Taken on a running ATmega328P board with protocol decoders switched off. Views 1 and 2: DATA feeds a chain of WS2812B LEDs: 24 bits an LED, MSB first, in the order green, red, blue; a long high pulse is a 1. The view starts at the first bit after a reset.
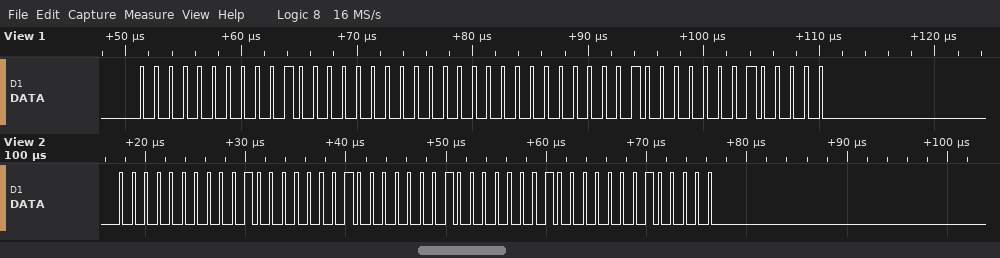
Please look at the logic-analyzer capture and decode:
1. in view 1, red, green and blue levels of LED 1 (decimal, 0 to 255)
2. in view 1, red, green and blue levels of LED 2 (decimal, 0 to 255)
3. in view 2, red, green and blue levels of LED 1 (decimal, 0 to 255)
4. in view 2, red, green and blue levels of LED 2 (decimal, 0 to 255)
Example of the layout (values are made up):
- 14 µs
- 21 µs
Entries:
- 32, 0, 0
- 32, 0, 32
- 32, 0, 32
- 32, 32, 32
